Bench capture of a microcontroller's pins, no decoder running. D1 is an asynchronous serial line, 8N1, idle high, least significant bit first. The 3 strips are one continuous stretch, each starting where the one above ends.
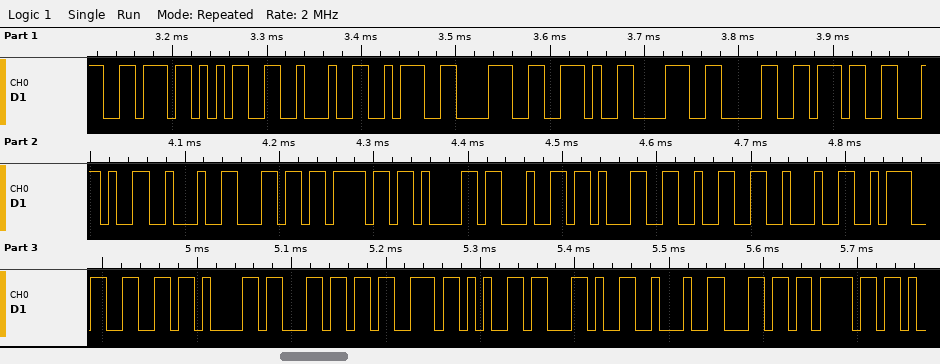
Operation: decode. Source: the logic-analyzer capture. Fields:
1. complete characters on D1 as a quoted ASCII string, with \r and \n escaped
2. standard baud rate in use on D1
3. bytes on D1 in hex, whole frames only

"v5\":8.807,\"load12\":false,\"lo"
115200 baud
76 35 22 3A 38 2E 38 30 37 2C 22 6C 6F 61 64 31 32 22 3A 66 61 6C 73 65 2C 22 6C 6F
